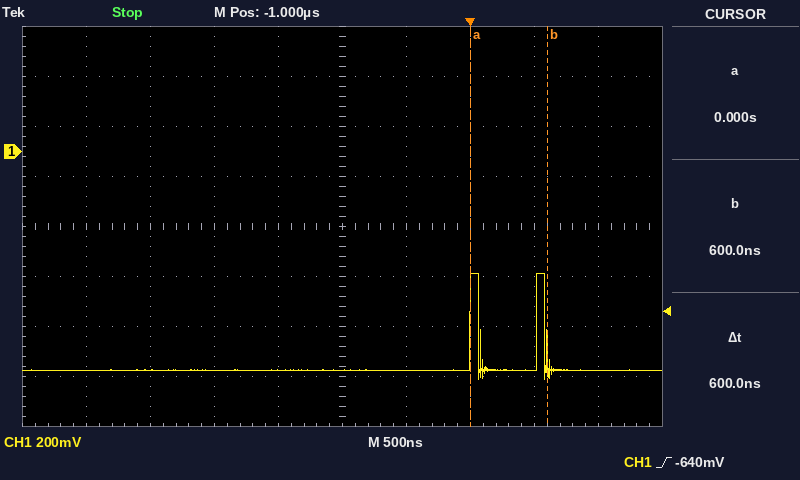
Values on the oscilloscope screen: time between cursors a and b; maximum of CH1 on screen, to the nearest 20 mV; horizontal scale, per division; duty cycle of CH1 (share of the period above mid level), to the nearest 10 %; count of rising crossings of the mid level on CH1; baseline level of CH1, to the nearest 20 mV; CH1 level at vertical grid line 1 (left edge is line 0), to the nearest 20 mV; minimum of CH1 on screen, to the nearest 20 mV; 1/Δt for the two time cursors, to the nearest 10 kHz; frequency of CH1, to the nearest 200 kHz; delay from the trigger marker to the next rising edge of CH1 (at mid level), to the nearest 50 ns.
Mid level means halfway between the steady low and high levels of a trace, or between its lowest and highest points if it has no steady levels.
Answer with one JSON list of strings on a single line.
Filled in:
["600 ns", "-480 mV", "500 ns", "10 %", "2", "-880 mV", "-880 mV", "-920 mV", "1.67 MHz", "2.0 MHz", "500 ns"]
